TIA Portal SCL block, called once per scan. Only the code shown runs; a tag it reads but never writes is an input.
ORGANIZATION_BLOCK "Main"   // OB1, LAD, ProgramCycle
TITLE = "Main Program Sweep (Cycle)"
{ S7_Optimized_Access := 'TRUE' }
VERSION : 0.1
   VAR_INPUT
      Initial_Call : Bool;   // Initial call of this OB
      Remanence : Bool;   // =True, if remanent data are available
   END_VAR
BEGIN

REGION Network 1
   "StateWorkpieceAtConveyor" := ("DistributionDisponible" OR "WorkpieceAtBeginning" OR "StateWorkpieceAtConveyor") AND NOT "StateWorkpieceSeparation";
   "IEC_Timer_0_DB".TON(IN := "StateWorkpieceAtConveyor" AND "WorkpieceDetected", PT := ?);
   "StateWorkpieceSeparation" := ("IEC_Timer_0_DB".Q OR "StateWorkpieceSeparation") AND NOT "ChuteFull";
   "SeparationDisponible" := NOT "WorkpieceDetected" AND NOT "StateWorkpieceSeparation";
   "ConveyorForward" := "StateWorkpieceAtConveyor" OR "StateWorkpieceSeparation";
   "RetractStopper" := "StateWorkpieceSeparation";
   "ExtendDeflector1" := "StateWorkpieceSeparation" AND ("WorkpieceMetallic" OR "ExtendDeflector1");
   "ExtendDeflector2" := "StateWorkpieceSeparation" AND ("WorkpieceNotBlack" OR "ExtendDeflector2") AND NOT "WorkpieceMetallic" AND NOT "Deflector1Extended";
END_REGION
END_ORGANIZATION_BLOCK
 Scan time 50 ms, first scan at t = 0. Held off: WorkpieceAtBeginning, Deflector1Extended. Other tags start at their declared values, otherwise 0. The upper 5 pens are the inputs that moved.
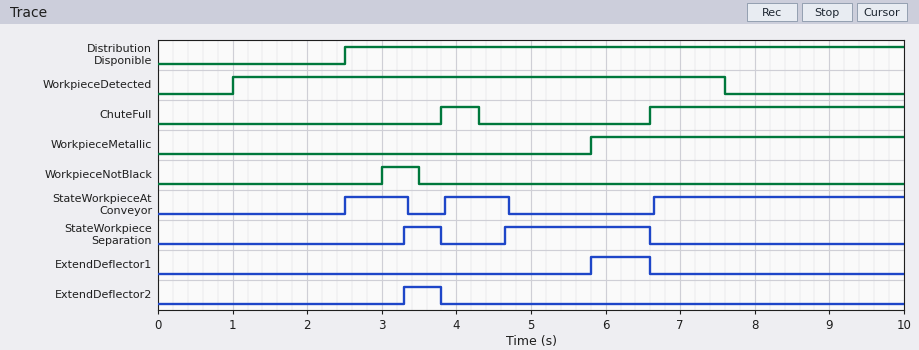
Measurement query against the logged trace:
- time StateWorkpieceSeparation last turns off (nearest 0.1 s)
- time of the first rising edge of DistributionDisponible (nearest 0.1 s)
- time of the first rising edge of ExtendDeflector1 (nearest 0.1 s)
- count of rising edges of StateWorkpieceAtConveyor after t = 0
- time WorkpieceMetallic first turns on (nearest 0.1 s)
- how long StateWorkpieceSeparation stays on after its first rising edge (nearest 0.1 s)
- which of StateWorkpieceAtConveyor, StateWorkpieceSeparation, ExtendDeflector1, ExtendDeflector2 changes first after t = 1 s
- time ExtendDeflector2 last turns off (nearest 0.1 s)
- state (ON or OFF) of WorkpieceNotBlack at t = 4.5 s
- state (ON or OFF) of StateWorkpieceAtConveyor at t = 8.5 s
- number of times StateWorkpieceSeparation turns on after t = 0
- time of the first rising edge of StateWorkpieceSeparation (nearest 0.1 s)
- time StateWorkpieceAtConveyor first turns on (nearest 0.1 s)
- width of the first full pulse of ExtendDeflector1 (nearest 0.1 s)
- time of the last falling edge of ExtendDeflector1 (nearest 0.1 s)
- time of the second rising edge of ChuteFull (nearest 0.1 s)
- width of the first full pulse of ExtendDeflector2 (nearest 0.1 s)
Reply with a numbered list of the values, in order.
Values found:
1. 6.6 s
2. 2.5 s
3. 5.8 s
4. 3
5. 5.8 s
6. 0.5 s
7. StateWorkpieceAtConveyor
8. 3.8 s
9. OFF
10. ON
11. 2
12. 3.3 s
13. 2.5 s
14. 0.8 s
15. 6.6 s
16. 6.6 s
17. 0.5 s
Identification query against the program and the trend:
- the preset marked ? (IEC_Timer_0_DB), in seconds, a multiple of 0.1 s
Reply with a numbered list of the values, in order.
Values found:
1. 0.8 s
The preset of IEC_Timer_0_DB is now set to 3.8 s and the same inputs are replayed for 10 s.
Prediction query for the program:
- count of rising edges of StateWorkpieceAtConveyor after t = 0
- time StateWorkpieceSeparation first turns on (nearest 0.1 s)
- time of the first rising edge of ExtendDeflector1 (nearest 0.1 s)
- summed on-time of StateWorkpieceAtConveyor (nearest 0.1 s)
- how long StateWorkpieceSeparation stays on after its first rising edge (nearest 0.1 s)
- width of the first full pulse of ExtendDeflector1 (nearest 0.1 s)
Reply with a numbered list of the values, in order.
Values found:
1. 2
2. 6.3 s
3. 6.3 s
4. 7.2 s
5. 0.3 s
6. 0.3 s
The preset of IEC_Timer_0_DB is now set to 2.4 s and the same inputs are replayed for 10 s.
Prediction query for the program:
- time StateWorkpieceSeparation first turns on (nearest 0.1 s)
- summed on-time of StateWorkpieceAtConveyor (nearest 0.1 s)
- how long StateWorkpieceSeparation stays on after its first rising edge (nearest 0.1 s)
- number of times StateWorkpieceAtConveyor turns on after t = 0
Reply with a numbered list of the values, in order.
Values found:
1. 4.9 s
2. 5.8 s
3. 1.7 s
4. 2
